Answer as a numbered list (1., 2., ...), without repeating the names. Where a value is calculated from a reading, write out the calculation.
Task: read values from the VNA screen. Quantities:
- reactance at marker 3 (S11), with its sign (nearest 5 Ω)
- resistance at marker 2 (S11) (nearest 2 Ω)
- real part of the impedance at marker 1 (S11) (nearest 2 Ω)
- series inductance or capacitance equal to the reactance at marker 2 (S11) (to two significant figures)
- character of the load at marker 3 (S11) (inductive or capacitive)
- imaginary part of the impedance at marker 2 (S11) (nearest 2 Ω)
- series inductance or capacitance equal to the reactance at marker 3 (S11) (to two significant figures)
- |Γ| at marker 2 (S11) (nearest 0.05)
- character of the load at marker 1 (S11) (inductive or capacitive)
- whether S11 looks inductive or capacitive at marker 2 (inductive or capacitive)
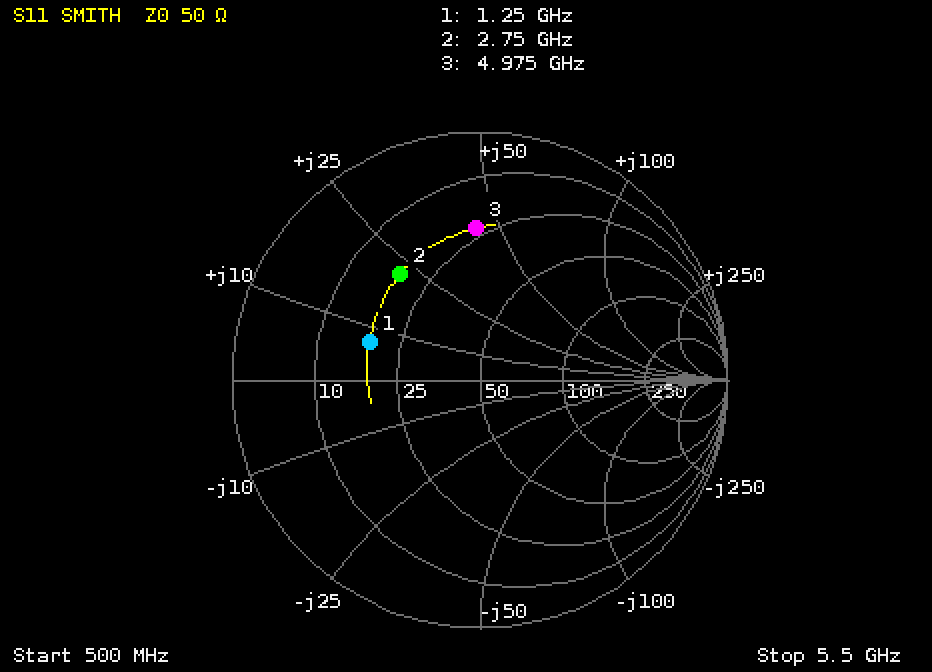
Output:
1. +45 Ω
2. 18 Ω
3. 18 Ω
4. L = 22 Ω/(2π × 2.75 GHz) ≈ 1.3 nH
5. inductive
6. +22 Ω
7. L = 45 Ω/(2π × 4.975 GHz) ≈ 1.4 nH
8. 0.55
9. inductive
10. inductive
